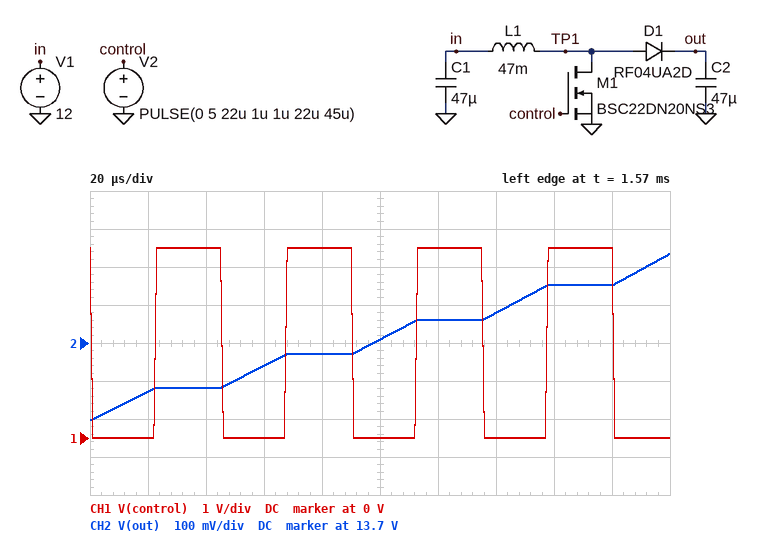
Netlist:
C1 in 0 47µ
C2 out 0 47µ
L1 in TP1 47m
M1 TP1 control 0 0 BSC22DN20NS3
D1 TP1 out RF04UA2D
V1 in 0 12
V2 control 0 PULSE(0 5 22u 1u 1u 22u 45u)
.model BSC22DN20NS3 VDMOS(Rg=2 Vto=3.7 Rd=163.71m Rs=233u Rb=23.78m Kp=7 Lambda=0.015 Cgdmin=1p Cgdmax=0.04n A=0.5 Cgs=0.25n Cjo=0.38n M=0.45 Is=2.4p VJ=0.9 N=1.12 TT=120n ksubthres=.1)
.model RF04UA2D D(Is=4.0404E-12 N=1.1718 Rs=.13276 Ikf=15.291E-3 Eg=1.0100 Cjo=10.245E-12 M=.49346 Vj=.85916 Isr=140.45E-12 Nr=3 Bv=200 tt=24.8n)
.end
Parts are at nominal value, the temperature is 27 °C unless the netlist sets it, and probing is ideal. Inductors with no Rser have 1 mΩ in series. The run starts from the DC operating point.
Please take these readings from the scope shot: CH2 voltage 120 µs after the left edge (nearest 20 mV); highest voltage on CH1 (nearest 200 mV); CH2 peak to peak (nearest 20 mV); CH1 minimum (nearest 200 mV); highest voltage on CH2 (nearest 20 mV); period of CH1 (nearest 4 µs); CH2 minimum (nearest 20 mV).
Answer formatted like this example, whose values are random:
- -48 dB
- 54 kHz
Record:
- 13.76 V
- 5.0 V
- 440 mV
- 0 V
- 13.94 V
- 44 µs
- 13.50 V
